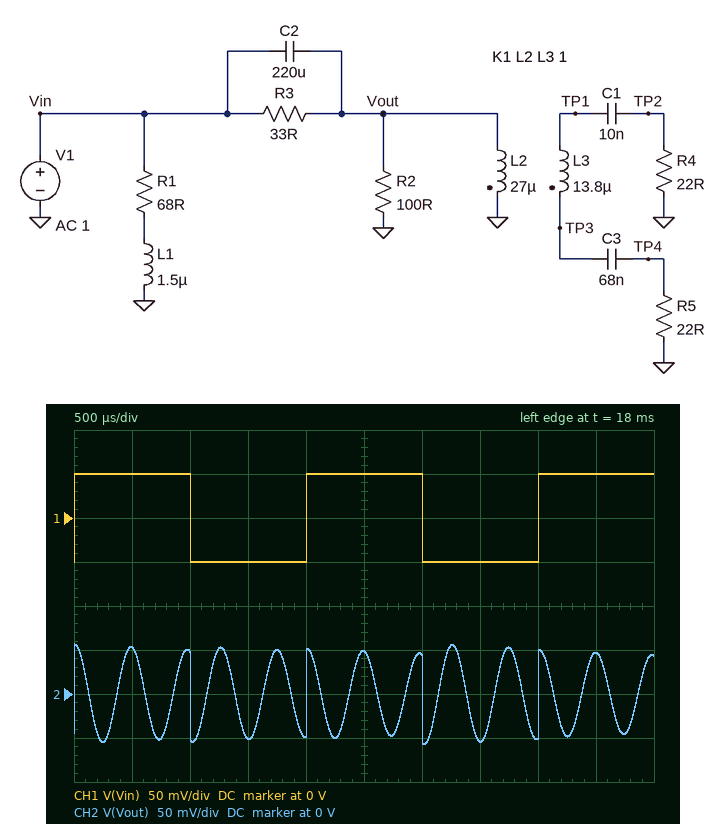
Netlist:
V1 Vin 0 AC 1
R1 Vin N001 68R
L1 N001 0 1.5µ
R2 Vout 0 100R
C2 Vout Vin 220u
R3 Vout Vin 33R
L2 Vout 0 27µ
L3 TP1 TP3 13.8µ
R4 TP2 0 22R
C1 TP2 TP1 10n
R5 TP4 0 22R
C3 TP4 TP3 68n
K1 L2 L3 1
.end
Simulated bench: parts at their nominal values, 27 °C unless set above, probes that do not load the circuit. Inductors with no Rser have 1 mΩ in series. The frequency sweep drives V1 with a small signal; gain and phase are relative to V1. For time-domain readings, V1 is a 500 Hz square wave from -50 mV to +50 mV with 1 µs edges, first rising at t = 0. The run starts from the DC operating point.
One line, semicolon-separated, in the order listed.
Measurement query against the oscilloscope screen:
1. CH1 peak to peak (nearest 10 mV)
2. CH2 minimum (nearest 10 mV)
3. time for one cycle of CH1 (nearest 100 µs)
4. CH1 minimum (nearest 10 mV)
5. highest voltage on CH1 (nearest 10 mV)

100 mV; -60 mV; 2.0 ms; -50 mV; 50 mV
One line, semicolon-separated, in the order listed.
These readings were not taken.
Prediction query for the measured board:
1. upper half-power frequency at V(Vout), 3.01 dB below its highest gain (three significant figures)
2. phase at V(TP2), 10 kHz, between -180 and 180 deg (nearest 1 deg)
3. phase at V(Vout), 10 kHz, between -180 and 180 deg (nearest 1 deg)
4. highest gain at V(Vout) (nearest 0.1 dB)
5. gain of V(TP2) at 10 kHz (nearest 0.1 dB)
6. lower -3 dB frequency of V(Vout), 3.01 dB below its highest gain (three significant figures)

2.08 kHz; 89 deg; 0 deg; 35.4 dB; -40.9 dB; 2.05 kHz
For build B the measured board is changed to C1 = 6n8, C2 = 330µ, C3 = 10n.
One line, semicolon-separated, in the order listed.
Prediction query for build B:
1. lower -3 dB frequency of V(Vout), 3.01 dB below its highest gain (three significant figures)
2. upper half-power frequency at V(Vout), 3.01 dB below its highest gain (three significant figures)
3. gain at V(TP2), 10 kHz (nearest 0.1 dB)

1.67 kHz; 1.70 kHz; -47.7 dB
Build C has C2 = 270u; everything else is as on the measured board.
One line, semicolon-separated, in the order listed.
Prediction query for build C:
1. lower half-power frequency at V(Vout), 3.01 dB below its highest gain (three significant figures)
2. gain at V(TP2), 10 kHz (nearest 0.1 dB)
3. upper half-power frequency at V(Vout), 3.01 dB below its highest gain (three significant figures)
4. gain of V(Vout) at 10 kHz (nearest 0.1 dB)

1.85 kHz; -41.0 dB; 1.88 kHz; 0.3 dB
